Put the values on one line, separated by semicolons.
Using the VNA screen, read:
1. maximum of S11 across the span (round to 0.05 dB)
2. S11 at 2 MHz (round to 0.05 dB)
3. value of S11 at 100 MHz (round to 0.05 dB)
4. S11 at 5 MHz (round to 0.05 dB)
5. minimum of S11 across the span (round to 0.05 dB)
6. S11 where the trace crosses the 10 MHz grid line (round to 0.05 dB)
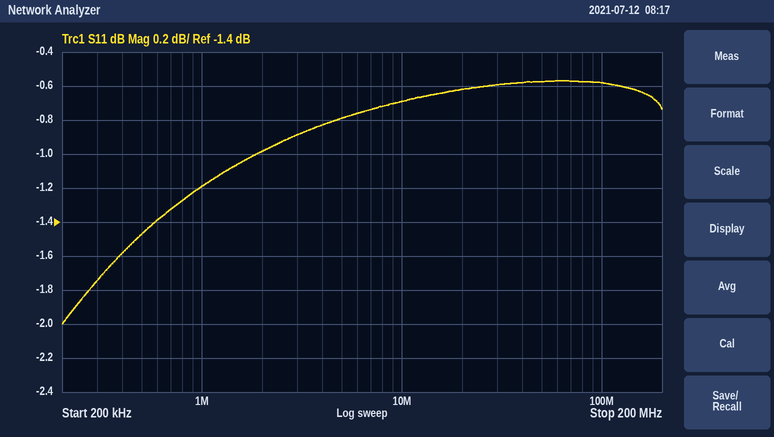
-0.55 dB; -1.00 dB; -0.60 dB; -0.80 dB; -2.00 dB; -0.70 dB
